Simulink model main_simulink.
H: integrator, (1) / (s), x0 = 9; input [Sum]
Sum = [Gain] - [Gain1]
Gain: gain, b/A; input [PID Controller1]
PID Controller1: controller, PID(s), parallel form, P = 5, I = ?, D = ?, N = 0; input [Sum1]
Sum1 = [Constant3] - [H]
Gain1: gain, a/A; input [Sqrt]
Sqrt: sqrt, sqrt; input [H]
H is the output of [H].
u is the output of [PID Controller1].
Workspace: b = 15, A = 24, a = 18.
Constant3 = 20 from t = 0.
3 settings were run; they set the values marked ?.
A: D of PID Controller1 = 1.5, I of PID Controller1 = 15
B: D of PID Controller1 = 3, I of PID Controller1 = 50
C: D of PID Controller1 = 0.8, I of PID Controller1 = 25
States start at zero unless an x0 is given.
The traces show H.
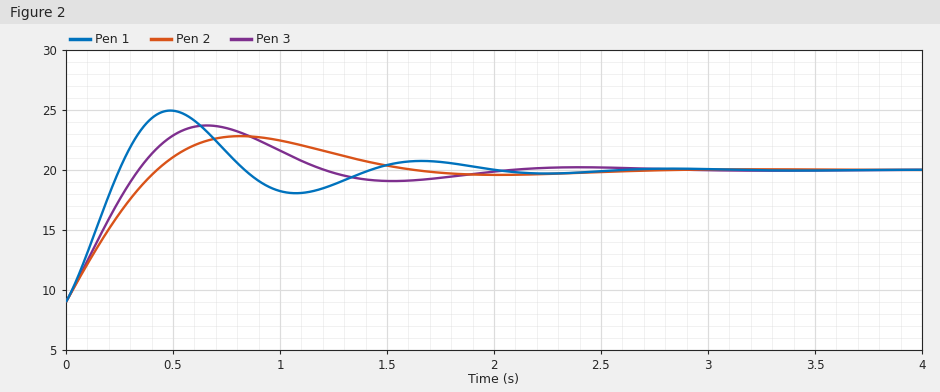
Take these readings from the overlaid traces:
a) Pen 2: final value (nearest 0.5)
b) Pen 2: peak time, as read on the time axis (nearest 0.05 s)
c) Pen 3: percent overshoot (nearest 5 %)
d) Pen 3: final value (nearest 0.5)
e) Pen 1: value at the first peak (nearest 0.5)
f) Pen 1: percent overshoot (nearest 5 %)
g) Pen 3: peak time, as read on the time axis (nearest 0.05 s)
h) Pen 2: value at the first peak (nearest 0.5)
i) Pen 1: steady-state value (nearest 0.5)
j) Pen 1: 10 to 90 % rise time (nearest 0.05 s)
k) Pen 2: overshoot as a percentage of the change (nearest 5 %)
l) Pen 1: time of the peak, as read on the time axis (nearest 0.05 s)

20.0
0.80 s
35 %
20.0
25.0
45 %
0.65 s
23.0
20.0
0.20 s
25 %
0.50 s
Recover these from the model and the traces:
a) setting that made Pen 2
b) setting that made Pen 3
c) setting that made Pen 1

A
C
B
